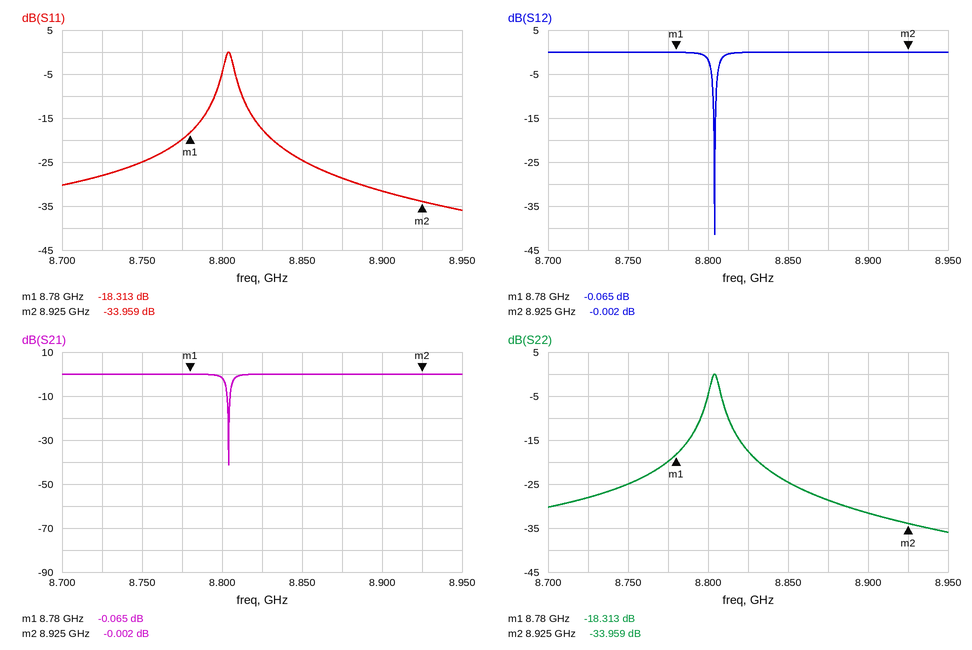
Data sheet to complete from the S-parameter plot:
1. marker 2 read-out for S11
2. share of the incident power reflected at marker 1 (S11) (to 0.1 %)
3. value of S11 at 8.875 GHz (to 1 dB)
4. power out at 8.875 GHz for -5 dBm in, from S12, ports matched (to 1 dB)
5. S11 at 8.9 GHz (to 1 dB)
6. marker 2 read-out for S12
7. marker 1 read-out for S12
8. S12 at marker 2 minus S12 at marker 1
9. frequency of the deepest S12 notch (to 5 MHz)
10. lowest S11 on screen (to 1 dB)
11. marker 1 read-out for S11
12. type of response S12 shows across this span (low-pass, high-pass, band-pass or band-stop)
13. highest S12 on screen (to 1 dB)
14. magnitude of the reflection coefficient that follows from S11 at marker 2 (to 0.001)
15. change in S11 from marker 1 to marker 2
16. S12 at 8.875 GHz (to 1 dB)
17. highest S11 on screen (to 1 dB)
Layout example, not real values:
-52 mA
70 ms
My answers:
-33.959 dB
1.5 %
-29 dB
-5 dBm
-32 dB
-0.002 dB
-0.065 dB
0.063 dB
8.805 GHz
-36 dB
-18.313 dB
band-stop
0 dB
0.020
-15.646 dB
0 dB
0 dB
